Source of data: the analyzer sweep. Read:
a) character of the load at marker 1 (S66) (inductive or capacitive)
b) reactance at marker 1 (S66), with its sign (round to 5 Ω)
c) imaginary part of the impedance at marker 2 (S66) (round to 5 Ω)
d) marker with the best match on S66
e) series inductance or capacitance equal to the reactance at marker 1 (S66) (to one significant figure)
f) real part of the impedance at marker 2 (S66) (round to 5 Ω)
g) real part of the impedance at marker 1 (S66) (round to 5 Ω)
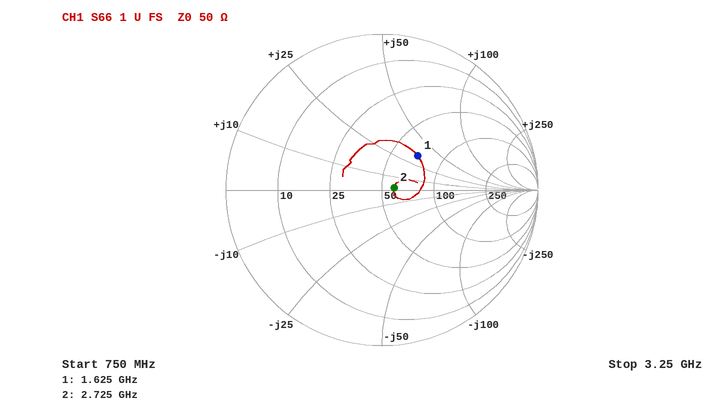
inductive
+35 Ω
0 Ω
marker 2
3 nH
60 Ω
70 Ω
